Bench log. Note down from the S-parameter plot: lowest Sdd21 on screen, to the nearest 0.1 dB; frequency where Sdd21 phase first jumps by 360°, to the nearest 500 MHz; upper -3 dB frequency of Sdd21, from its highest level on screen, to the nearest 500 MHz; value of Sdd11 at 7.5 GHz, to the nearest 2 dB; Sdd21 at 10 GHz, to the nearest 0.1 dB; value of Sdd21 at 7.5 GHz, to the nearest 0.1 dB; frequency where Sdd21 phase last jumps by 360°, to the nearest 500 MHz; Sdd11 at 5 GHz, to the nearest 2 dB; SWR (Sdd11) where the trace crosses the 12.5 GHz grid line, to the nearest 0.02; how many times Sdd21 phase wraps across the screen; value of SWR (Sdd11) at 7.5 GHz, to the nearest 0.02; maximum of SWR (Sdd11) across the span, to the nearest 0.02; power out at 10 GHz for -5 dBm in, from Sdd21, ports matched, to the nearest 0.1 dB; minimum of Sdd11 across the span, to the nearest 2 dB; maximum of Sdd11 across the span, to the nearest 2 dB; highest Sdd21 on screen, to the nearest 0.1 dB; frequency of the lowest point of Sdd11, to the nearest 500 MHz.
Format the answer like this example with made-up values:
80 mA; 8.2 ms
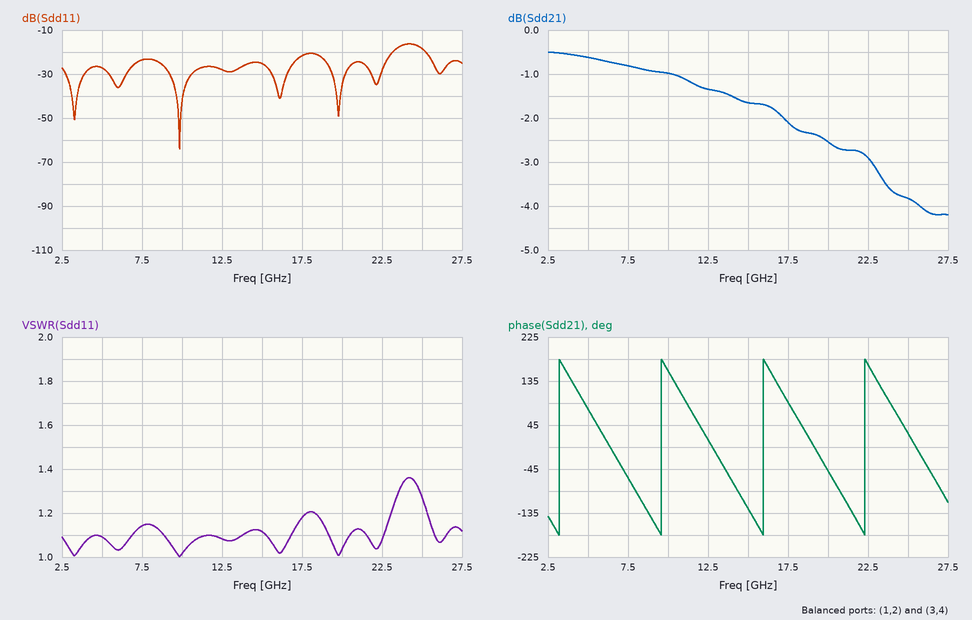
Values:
-4.2 dB; 3.0 GHz; 23.5 GHz; -24 dB; -1.0 dB; -0.8 dB; 22.5 GHz; -28 dB; 1.08; 4; 1.14; 1.36; -6.0 dBm; -64 dB; -16 dB; -0.5 dB; 10.0 GHz
